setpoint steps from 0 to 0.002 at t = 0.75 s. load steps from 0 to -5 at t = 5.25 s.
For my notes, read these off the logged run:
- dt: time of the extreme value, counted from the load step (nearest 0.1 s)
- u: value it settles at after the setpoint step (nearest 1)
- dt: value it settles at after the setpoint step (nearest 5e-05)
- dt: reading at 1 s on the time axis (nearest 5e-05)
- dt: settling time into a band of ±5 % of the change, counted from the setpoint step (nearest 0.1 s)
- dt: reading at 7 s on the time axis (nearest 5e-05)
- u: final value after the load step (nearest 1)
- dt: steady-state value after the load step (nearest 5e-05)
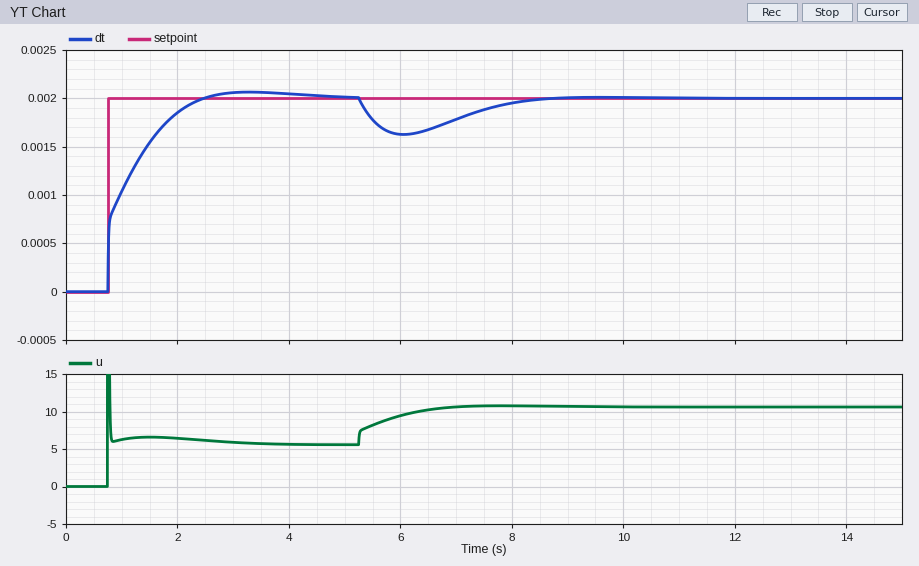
0.8 s
6
0.00200
0.00105
1.4 s
0.00180
11
0.00200
